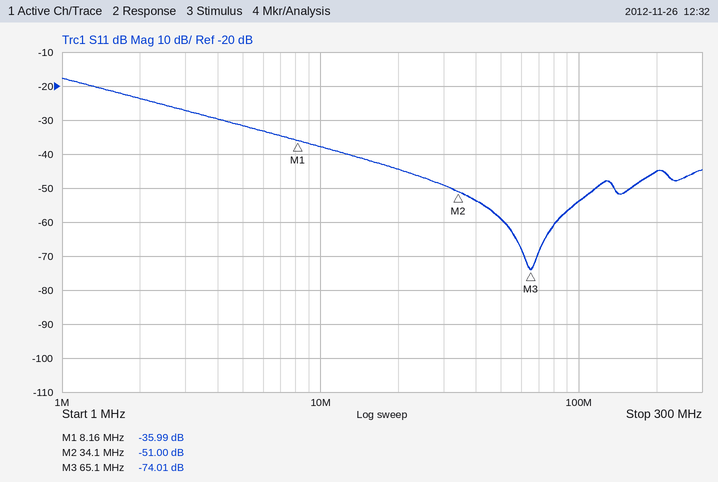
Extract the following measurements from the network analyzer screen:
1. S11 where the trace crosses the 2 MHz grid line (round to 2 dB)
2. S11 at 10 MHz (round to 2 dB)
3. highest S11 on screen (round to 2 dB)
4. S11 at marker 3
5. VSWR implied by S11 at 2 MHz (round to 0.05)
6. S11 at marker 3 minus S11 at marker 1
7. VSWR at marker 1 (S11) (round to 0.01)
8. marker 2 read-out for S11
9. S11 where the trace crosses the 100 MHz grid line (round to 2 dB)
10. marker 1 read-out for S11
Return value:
-24 dB
-38 dB
-18 dB
-74.01 dB
1.15
-38.02 dB
1.03
-51.00 dB
-54 dB
-35.99 dB
